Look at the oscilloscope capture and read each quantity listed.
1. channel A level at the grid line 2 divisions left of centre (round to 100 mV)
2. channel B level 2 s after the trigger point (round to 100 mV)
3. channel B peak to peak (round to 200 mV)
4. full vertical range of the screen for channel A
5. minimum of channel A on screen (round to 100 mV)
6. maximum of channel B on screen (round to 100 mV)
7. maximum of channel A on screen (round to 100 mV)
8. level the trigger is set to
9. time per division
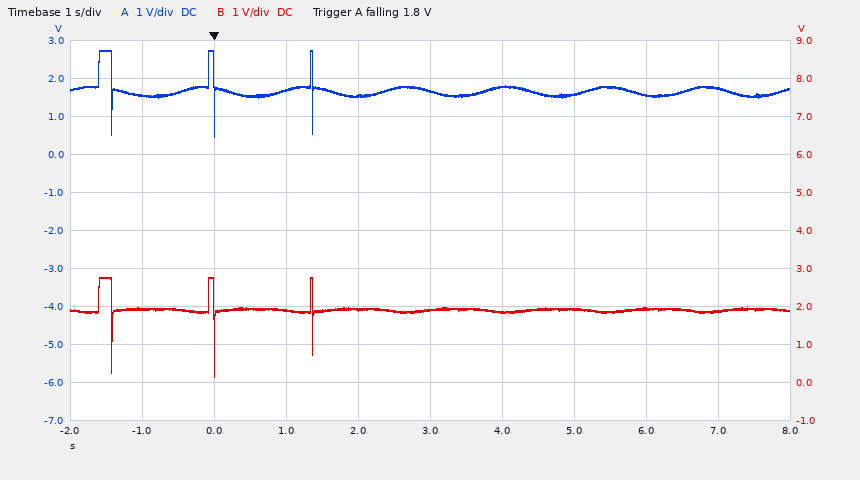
1.7 V
1.9 V
2.6 V
10 V
500 mV
2.8 V
2.7 V
1.8 V
1 s
